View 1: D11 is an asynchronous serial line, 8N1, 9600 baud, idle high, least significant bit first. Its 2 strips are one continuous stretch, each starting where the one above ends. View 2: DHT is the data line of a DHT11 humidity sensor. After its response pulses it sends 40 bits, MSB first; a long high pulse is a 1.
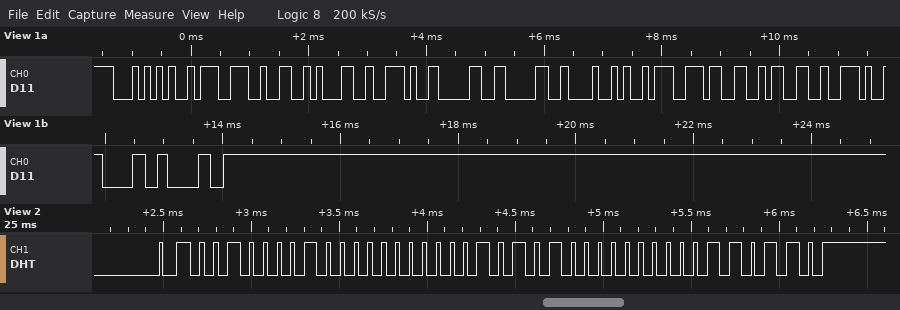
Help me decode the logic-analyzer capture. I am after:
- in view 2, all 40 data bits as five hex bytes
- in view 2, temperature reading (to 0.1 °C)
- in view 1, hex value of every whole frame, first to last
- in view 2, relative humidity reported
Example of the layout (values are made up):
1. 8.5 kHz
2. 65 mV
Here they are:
1. 21 00 15 00 36
2. 21.0 °C
3. 54 3A 32 31 2E 30 30 48 3A 33 33 2E 30 30
4. 33 %
